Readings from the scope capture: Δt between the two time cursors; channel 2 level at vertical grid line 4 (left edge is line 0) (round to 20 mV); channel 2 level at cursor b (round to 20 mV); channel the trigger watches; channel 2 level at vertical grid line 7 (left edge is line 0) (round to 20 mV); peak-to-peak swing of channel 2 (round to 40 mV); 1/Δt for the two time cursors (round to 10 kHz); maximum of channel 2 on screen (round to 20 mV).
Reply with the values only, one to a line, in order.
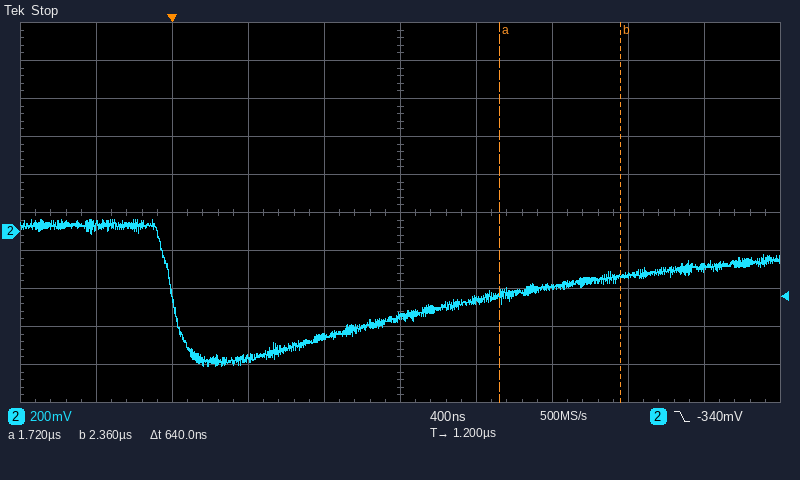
640 ns
-560 mV
-240 mV
channel 2
-300 mV
760 mV
1.56 MHz
60 mV
